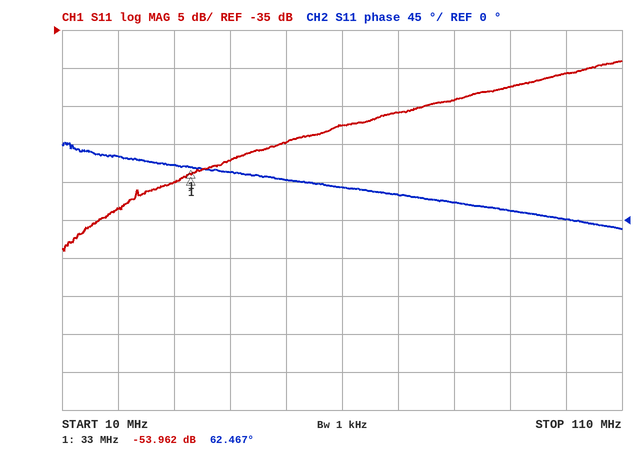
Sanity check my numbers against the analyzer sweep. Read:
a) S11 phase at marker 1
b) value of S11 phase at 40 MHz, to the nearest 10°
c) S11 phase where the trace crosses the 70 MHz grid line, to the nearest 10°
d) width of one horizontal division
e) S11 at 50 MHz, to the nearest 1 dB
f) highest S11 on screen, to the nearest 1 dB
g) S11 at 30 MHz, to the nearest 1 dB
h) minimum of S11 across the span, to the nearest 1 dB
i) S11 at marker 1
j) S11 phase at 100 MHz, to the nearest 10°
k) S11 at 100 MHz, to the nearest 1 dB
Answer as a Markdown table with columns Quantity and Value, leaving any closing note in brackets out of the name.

| Quantity | Value |
|---|---|
| S11 phase at marker 1 | 62.467° |
| value of S11 phase at 40 MHz, to the nearest 10° | 60° |
| S11 phase where the trace crosses the 70 MHz grid line, to the nearest 10° | 30° |
| width of one horizontal division | 10 MHz |
| S11 at 50 MHz, to the nearest 1 dB | -50 dB |
| highest S11 on screen, to the nearest 1 dB | -39 dB |
| S11 at 30 MHz, to the nearest 1 dB | -55 dB |
| minimum of S11 across the span, to the nearest 1 dB | -64 dB |
| S11 at marker 1 | -53.962 dB |
| S11 phase at 100 MHz, to the nearest 10° | 0° |
| S11 at 100 MHz, to the nearest 1 dB | -41 dB |
